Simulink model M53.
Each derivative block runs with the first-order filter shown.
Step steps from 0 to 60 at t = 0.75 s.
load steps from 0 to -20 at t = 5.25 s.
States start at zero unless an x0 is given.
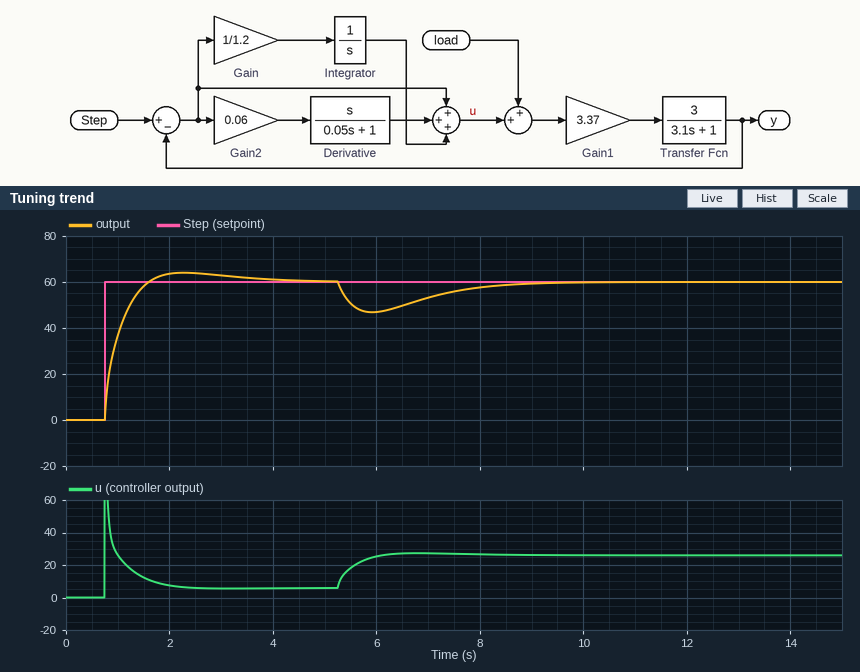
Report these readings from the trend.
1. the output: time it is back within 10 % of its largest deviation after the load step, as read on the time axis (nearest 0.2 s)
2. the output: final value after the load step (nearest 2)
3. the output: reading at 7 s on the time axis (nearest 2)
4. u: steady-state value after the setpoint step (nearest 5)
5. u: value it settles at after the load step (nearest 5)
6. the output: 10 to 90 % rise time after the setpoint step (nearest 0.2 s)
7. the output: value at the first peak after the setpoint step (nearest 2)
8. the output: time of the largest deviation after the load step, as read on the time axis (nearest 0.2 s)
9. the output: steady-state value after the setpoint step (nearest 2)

8.4 s
60
54
5
25
0.6 s
64
6.0 s
60
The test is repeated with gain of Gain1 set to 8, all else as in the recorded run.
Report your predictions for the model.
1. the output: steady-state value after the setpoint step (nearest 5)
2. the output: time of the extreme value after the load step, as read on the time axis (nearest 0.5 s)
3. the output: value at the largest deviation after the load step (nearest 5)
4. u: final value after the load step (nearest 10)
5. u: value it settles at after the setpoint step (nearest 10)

60
5.5 s
45
20
0
